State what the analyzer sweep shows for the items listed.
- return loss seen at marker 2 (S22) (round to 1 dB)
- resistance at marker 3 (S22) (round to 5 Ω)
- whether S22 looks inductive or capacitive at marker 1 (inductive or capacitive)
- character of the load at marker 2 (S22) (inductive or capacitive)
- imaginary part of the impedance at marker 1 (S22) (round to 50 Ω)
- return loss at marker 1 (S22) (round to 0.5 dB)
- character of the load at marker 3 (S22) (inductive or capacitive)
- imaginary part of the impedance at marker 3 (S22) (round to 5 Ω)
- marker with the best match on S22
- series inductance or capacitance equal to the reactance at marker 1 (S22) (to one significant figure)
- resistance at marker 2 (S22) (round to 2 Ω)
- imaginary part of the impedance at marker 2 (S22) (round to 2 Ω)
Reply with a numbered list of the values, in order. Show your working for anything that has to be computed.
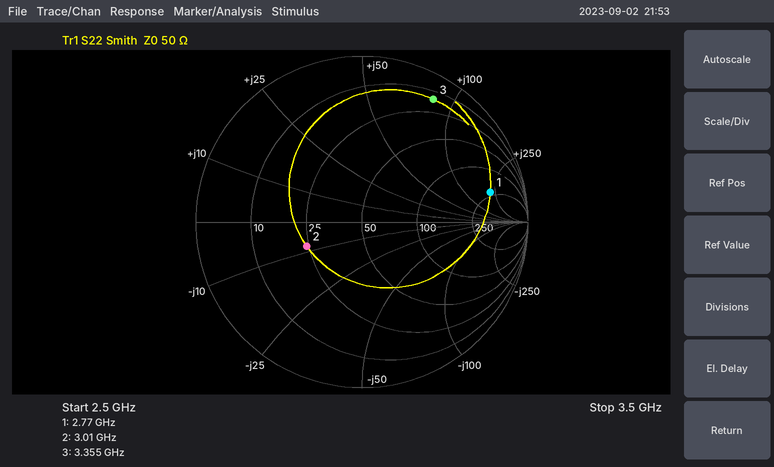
1. 9 dB
2. 15 Ω
3. inductive
4. capacitive
5. +200 Ω
6. 2.0 dB
7. inductive
8. +85 Ω
9. marker 2
10. L = 200 Ω/(2π × 2.77 GHz) ≈ 11.5 nH, so 10 nH to one significant figure
11. 24 Ω
12. -8 Ω
